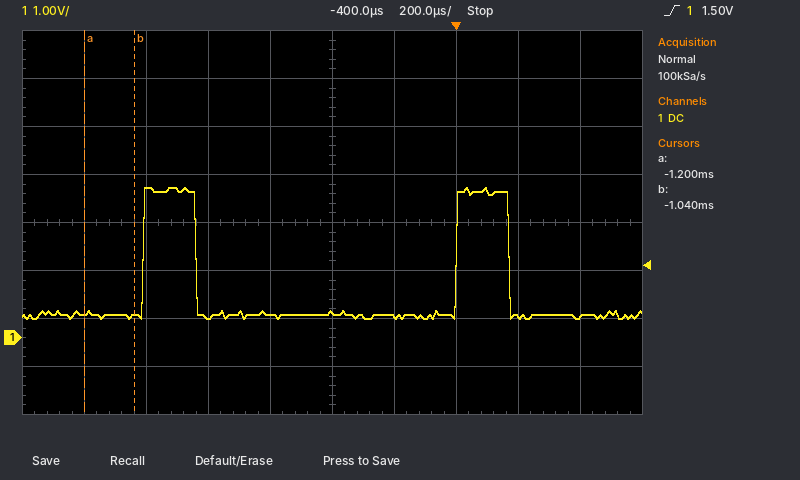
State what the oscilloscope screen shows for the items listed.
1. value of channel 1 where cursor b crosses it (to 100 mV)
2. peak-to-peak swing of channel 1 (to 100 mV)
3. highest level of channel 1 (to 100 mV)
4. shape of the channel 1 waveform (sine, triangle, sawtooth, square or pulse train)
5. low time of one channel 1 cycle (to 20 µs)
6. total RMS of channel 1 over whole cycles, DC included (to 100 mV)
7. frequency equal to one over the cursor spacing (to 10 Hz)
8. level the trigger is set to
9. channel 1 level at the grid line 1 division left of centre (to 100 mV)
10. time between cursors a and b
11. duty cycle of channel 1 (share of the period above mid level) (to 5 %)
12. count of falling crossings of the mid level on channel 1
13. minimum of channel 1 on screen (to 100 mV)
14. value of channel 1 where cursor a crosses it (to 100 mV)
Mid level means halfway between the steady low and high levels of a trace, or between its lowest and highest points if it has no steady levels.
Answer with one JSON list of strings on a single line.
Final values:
["500 mV", "2.7 V", "3.1 V", "pulse train", "840 µs", "1.3 V", "6.25 kHz", "1.50 V", "500 mV", "160 µs", "15 %", "2", "400 mV", "500 mV"]
